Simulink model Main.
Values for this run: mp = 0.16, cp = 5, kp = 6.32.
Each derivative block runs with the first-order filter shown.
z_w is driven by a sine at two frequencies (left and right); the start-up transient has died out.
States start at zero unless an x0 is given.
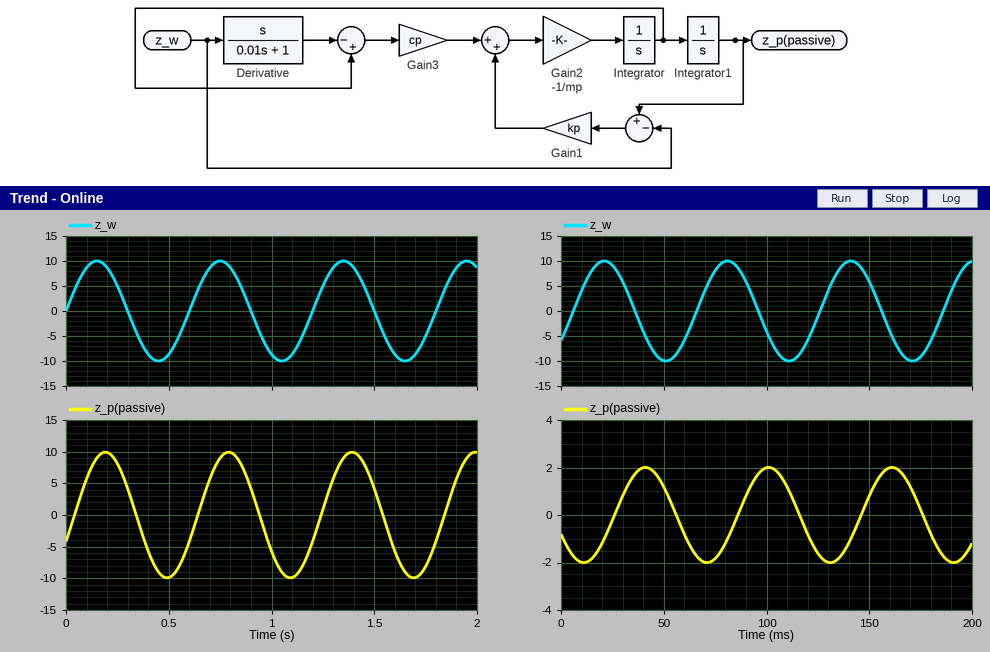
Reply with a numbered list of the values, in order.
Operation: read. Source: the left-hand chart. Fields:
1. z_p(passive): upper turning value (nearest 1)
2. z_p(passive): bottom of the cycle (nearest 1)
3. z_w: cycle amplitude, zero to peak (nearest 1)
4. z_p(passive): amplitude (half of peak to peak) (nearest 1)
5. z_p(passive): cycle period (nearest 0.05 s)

1. 10
2. -10
3. 10
4. 10
5. 0.60 s
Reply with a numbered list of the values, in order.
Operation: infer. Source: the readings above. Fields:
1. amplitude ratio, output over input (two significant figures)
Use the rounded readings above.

1. 1.0
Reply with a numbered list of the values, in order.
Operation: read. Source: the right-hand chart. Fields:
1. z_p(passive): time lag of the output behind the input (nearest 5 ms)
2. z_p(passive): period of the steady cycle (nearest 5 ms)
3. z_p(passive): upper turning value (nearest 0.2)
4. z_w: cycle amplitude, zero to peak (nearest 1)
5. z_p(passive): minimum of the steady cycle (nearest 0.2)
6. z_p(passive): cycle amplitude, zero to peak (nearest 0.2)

1. 20 ms
2. 60 ms
3. 2.0
4. 10
5. -2.0
6. 2.0
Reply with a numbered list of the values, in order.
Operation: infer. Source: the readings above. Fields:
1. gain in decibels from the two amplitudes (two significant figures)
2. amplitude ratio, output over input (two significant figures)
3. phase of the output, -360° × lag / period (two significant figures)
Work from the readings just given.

1. -14 dB
2. 0.20
3. -120°
